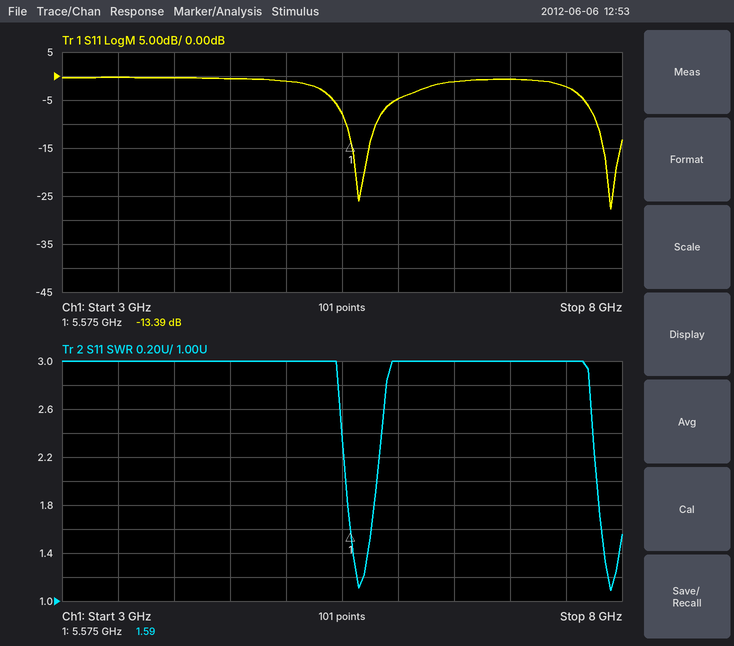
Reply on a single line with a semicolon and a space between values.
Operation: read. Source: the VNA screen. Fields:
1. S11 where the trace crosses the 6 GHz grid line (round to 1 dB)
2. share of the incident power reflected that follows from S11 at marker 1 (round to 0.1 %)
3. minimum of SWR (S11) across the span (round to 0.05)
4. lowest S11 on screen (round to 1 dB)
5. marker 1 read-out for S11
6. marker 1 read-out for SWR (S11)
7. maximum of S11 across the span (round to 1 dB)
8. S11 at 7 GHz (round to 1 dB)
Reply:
-5 dB; 4.6 %; 1.10; -28 dB; -13.39 dB; 1.59; 0 dB; -1 dB
